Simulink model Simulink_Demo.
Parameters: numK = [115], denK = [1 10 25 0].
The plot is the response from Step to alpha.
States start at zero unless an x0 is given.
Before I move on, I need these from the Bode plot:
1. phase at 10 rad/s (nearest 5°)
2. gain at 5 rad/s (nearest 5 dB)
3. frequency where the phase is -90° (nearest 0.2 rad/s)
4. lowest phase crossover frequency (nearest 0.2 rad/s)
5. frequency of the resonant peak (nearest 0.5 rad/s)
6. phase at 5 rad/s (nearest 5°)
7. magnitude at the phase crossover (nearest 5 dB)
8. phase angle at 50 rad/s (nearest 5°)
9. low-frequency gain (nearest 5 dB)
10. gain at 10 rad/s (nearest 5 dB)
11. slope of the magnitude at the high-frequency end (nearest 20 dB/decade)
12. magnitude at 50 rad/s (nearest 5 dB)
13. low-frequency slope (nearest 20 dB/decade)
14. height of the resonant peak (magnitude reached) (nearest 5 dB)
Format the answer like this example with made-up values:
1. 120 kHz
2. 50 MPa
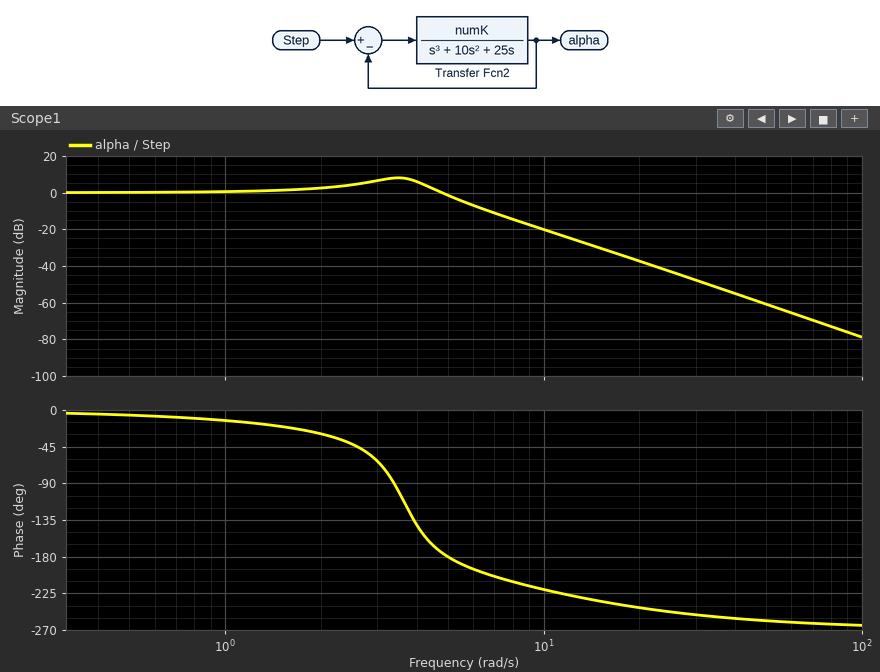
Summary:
1. -220°
2. 0 dB
3. 3.4 rad/s
4. 5.0 rad/s
5. 3.5 rad/s
6. -180°
7. 0 dB
8. -260°
9. 0 dB
10. -20 dB
11. -60 dB/decade
12. -60 dB
13. 0 dB/decade
14. 10 dB
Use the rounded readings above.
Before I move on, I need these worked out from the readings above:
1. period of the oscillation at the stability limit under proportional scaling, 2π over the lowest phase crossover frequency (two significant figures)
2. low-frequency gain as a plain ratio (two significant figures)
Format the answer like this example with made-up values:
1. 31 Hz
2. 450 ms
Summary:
1. 1.3 s
2. 1.0
